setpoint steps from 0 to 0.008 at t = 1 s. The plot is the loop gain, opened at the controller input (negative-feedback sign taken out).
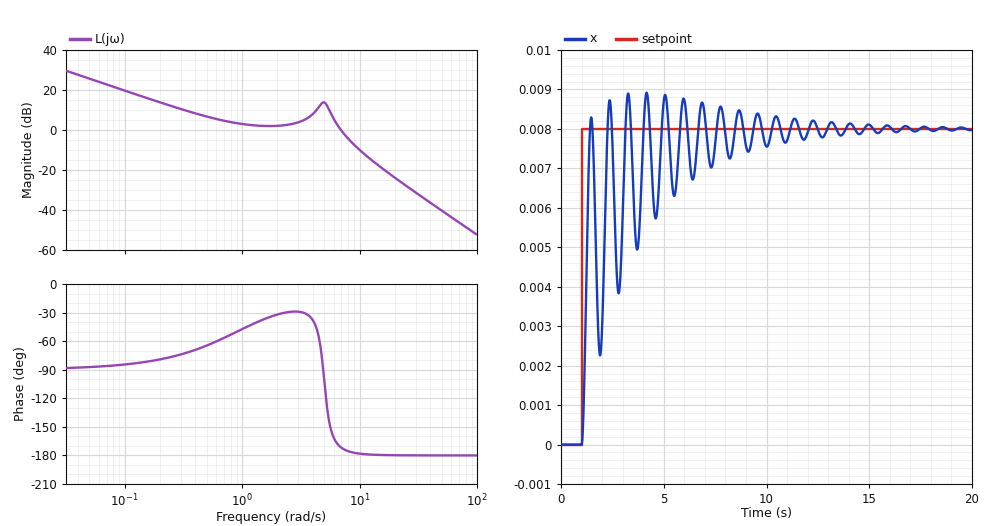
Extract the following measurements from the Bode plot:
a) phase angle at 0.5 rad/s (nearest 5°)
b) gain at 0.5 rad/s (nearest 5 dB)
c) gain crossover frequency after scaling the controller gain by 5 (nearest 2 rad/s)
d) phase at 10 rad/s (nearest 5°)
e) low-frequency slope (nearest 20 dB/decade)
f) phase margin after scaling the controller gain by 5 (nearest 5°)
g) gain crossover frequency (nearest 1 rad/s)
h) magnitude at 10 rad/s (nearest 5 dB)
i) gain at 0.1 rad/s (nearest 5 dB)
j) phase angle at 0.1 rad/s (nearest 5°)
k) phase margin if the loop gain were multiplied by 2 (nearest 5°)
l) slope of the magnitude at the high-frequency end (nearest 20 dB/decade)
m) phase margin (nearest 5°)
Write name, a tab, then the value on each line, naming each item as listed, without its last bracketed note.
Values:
phase angle at 0.5 rad/s	-65°
gain at 0.5 rad/s	5 dB
gain crossover frequency after scaling the controller gain by 5	12 rad/s
phase at 10 rad/s	-180°
low-frequency slope	-20 dB/decade
phase margin after scaling the controller gain by 5	0°
gain crossover frequency	7 rad/s
magnitude at 10 rad/s	-10 dB
gain at 0.1 rad/s	20 dB
phase angle at 0.1 rad/s	-85°
phase margin if the loop gain were multiplied by 2	5°
slope of the magnitude at the high-frequency end	-40 dB/decade
phase margin	10°
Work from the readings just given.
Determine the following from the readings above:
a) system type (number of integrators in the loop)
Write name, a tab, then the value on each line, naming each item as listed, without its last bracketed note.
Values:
system type	1
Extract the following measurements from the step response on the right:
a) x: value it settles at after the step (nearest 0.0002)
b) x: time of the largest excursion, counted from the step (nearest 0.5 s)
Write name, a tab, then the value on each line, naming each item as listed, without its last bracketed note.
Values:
x: value it settles at after the step	0.0080
x: time of the largest excursion, counted from the step	3.0 s
